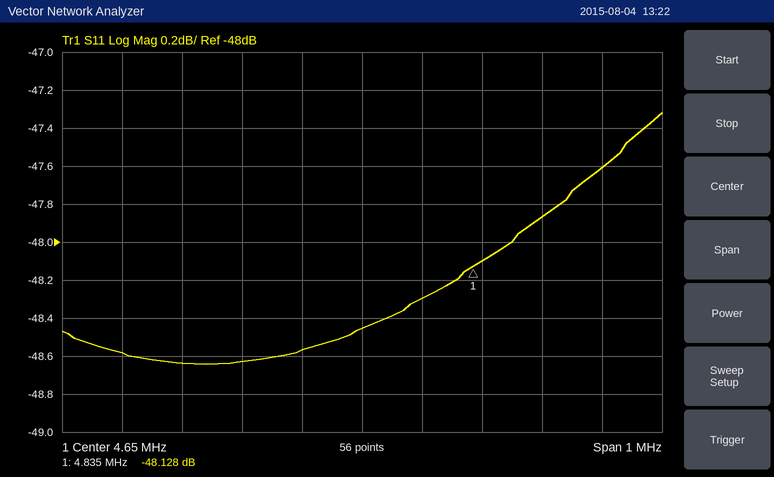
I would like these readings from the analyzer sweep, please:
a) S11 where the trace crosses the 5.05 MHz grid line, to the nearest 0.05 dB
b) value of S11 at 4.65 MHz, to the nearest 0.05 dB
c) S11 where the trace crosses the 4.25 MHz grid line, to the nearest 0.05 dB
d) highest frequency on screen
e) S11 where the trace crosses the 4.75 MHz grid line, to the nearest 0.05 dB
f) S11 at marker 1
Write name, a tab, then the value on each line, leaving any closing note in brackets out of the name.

S11 where the trace crosses the 5.05 MHz grid line, to the nearest 0.05 dB	-47.60 dB
value of S11 at 4.65 MHz, to the nearest 0.05 dB	-48.45 dB
S11 where the trace crosses the 4.25 MHz grid line, to the nearest 0.05 dB	-48.60 dB
highest frequency on screen	5.15 MHz
S11 where the trace crosses the 4.75 MHz grid line, to the nearest 0.05 dB	-48.30 dB
S11 at marker 1	-48.128 dB
